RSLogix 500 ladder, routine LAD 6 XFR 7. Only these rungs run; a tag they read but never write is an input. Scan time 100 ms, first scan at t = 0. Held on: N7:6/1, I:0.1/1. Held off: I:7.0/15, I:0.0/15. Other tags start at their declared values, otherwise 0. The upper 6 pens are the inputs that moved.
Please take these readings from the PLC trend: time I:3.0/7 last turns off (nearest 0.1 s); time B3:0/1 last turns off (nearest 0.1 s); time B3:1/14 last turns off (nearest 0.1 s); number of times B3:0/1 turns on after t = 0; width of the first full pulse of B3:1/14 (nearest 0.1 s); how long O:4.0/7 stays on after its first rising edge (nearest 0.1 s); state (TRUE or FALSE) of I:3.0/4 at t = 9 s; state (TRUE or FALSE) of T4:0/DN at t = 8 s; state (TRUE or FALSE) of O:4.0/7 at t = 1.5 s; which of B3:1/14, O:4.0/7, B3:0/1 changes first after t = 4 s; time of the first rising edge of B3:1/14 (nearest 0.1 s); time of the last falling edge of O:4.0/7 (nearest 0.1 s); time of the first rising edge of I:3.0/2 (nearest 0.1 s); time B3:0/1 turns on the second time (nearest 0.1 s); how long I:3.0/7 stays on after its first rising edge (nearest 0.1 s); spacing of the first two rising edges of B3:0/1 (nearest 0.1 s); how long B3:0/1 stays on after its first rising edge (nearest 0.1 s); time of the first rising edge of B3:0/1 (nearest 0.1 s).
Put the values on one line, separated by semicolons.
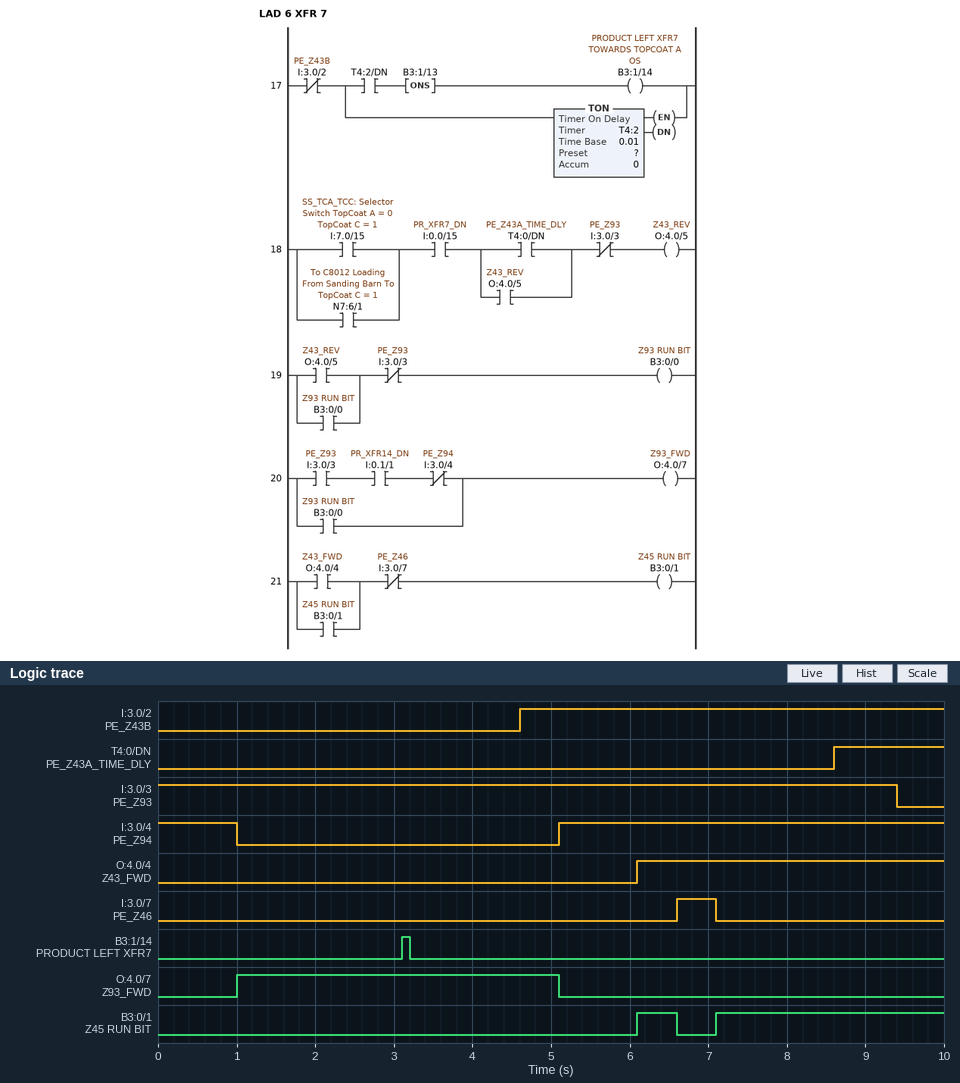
7.1 s; 6.6 s; 3.2 s; 2; 0.1 s; 4.1 s; TRUE; FALSE; TRUE; O:4.0/7; 3.1 s; 5.1 s; 4.6 s; 7.1 s; 0.5 s; 1.0 s; 0.5 s; 6.1 s
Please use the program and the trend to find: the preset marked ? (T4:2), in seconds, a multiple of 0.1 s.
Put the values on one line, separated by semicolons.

3.0 s
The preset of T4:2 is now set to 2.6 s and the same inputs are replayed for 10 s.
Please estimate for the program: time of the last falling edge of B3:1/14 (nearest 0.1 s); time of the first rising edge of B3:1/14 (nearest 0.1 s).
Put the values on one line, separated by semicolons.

2.8 s; 2.7 s
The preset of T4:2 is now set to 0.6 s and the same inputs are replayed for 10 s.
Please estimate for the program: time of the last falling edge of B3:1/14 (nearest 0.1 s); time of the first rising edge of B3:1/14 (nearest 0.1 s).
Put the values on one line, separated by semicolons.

0.8 s; 0.7 s
